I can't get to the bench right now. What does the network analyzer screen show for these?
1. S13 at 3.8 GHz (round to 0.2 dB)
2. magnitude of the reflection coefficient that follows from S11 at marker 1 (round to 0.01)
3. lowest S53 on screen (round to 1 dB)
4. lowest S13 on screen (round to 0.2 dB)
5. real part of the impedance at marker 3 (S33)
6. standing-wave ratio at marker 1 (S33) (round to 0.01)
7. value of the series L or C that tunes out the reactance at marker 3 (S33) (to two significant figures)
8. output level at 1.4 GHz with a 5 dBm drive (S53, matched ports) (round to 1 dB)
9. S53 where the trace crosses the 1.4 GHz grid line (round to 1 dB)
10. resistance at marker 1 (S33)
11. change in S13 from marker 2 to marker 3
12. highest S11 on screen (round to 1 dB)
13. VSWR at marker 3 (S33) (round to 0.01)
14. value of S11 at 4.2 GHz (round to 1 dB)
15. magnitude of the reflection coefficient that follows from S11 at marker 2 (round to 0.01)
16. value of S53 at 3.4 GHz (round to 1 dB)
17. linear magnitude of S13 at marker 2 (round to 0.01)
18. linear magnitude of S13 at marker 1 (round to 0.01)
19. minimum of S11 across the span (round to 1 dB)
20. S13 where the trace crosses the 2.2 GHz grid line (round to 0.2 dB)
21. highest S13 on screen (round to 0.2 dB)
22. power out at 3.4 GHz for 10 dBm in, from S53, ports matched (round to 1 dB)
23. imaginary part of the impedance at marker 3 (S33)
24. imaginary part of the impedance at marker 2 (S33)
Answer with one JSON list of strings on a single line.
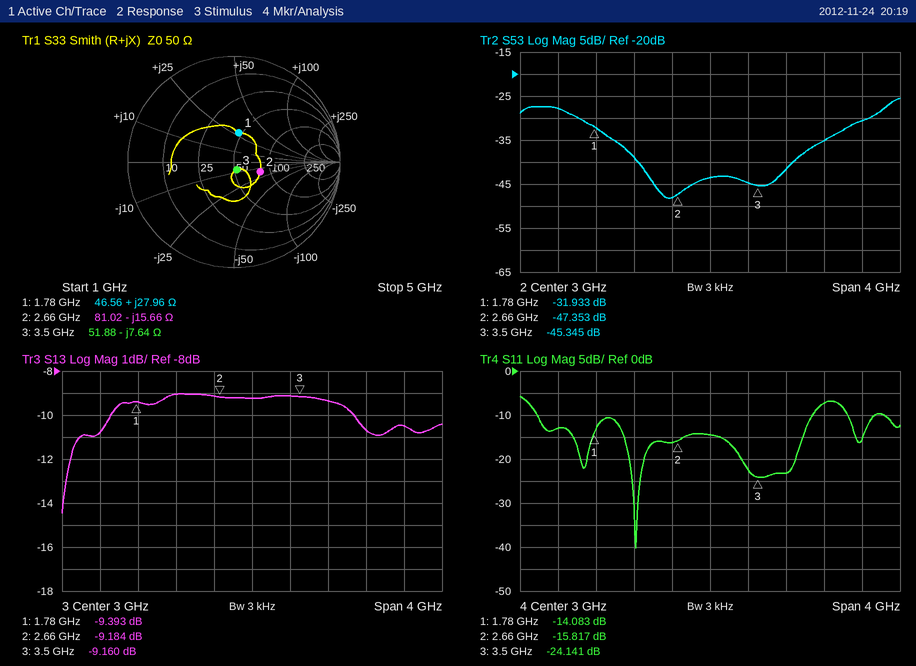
["-9.4 dB", "0.20", "-48 dB", "-14.4 dB", "51.88 Ω", "1.78", "350 pH", "-23 dBm", "-28 dB", "46.56 Ω", "0.024 dB", "-6 dB", "1.17", "-7 dB", "0.16", "-45 dB", "0.35", "0.34", "-40 dB", "-9.0 dB", "-9.0 dB", "-35 dBm", "-7.64 Ω", "-15.66 Ω"]
